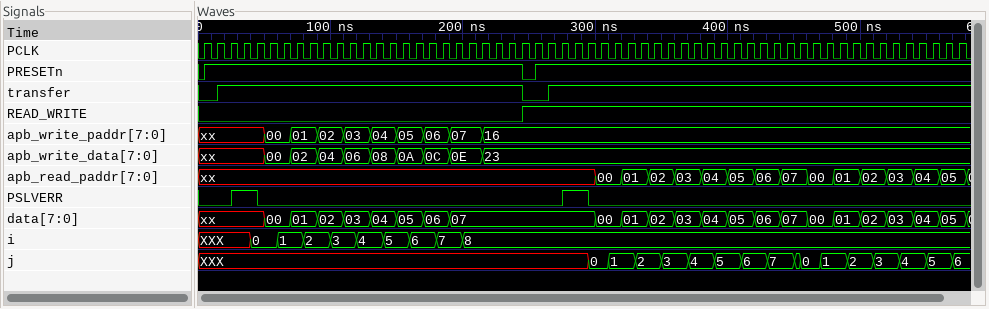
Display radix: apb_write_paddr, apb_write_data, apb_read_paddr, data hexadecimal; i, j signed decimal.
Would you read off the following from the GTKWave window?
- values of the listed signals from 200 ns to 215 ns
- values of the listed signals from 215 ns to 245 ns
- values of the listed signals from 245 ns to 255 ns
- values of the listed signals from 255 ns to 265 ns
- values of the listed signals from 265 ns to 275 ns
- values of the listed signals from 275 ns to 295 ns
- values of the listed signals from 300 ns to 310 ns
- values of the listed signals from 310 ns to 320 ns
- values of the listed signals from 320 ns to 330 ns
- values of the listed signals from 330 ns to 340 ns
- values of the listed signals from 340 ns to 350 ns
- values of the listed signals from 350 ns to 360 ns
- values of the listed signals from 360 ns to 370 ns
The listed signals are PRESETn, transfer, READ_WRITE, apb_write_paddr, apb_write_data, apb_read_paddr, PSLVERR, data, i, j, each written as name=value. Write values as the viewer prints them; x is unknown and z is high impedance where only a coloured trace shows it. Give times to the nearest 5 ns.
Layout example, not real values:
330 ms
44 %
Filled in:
PRESETn=1, transfer=1, READ_WRITE=0, apb_write_paddr=07, apb_write_data=0E, apb_read_paddr=xx, PSLVERR=0, data=07, i=8, j=XXX
PRESETn=1, transfer=1, READ_WRITE=0, apb_write_paddr=16, apb_write_data=23, apb_read_paddr=xx, PSLVERR=0, data=07, i=8, j=XXX
PRESETn=0, transfer=0, READ_WRITE=1, apb_write_paddr=16, apb_write_data=23, apb_read_paddr=xx, PSLVERR=0, data=07, i=8, j=XXX
PRESETn=1, transfer=0, READ_WRITE=1, apb_write_paddr=16, apb_write_data=23, apb_read_paddr=xx, PSLVERR=0, data=07, i=8, j=XXX
PRESETn=1, transfer=1, READ_WRITE=1, apb_write_paddr=16, apb_write_data=23, apb_read_paddr=xx, PSLVERR=0, data=07, i=8, j=XXX
PRESETn=1, transfer=1, READ_WRITE=1, apb_write_paddr=16, apb_write_data=23, apb_read_paddr=xx, PSLVERR=1, data=07, i=8, j=XXX
PRESETn=1, transfer=1, READ_WRITE=1, apb_write_paddr=16, apb_write_data=23, apb_read_paddr=00, PSLVERR=0, data=00, i=8, j=0
PRESETn=1, transfer=1, READ_WRITE=1, apb_write_paddr=16, apb_write_data=23, apb_read_paddr=00, PSLVERR=0, data=00, i=8, j=1
PRESETn=1, transfer=1, READ_WRITE=1, apb_write_paddr=16, apb_write_data=23, apb_read_paddr=01, PSLVERR=0, data=01, i=8, j=1
PRESETn=1, transfer=1, READ_WRITE=1, apb_write_paddr=16, apb_write_data=23, apb_read_paddr=01, PSLVERR=0, data=01, i=8, j=2
PRESETn=1, transfer=1, READ_WRITE=1, apb_write_paddr=16, apb_write_data=23, apb_read_paddr=02, PSLVERR=0, data=02, i=8, j=2
PRESETn=1, transfer=1, READ_WRITE=1, apb_write_paddr=16, apb_write_data=23, apb_read_paddr=02, PSLVERR=0, data=02, i=8, j=3
PRESETn=1, transfer=1, READ_WRITE=1, apb_write_paddr=16, apb_write_data=23, apb_read_paddr=03, PSLVERR=0, data=03, i=8, j=3
